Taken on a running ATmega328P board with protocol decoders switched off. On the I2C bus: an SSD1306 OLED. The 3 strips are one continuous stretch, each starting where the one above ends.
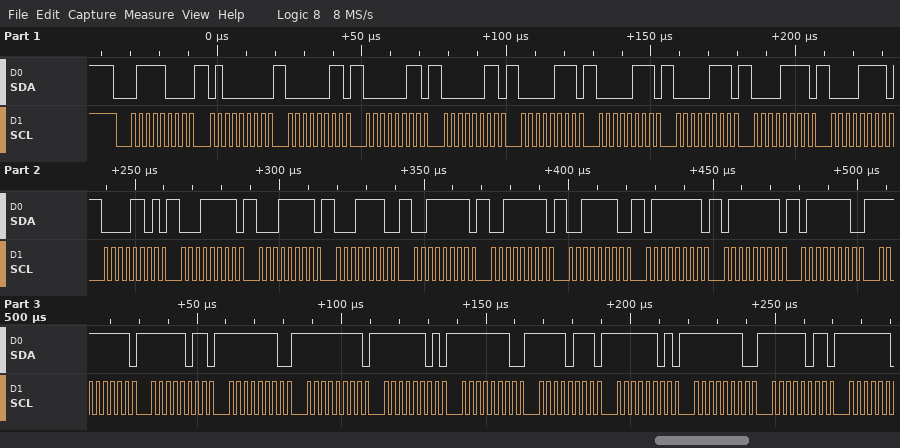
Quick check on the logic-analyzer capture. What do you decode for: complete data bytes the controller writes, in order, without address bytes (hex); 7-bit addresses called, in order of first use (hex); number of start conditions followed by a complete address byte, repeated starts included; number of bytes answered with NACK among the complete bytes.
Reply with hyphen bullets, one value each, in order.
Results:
- 40 03 03 03 07 07 07 0F 0F 0D 1F 1F 1E 3F 3F 3E 7F 7F 7E FF FB FE FF FD FE F7 FD FE FB
- 0x3C
- 1
- 0
